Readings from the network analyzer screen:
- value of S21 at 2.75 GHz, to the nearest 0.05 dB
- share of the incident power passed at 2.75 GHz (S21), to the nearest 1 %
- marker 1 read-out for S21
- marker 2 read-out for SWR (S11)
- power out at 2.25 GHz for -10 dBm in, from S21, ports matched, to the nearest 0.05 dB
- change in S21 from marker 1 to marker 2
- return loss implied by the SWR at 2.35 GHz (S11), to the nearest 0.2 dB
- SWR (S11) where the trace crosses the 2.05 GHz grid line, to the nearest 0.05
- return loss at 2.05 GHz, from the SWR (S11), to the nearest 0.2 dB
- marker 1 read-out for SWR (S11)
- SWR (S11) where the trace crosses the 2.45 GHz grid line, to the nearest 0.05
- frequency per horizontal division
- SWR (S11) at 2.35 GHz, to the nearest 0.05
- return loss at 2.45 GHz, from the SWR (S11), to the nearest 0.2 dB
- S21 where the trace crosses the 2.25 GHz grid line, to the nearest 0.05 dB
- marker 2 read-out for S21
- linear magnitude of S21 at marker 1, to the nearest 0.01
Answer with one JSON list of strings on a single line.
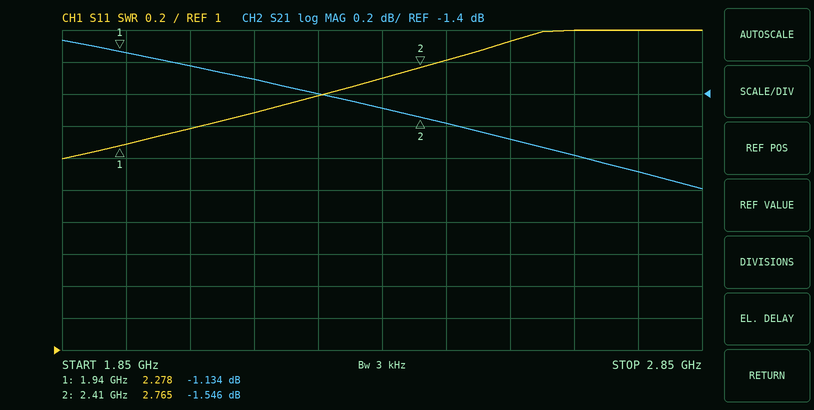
["-1.90 dB", "65 %", "-1.134 dB", "2.765", "-11.40 dBm", "-0.412 dB", "6.8 dB", "2.40", "7.8 dB", "2.278", "2.80", "100 MHz", "2.70", "6.4 dB", "-1.40 dB", "-1.546 dB", "0.88"]
